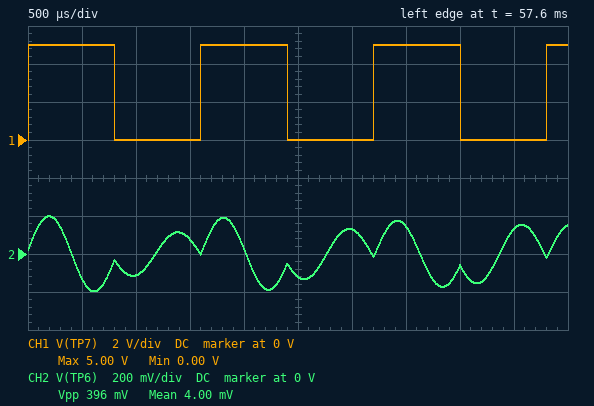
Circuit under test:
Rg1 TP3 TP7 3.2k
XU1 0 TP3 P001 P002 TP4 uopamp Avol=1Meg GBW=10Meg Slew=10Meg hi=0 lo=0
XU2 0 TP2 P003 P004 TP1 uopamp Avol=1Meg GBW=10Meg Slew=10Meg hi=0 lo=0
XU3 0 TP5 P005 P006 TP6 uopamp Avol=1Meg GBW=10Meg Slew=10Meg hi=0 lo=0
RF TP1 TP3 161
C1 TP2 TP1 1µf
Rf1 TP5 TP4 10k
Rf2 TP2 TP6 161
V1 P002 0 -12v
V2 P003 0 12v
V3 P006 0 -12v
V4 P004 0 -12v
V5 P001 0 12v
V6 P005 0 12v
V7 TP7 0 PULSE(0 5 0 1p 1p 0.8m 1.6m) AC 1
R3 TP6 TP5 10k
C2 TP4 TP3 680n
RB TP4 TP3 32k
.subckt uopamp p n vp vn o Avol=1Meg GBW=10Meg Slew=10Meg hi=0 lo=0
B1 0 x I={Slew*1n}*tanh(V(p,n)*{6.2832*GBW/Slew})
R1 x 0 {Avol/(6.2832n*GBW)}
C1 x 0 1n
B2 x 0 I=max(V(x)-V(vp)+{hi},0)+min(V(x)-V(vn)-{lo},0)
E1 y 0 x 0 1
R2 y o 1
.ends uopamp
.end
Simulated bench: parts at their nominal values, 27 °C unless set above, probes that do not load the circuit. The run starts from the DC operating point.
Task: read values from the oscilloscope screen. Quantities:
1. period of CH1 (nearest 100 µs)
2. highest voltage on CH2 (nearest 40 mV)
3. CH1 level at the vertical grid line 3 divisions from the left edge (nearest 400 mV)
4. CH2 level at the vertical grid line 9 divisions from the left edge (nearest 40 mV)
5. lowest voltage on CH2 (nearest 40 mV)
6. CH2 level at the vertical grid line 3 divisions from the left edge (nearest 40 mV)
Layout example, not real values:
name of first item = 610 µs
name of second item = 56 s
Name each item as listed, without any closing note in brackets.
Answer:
period of CH1 = 1.6 ms
highest voltage on CH2 = 200 mV
CH1 level at the vertical grid line 3 divisions from the left edge = 0 V
CH2 level at the vertical grid line 9 divisions from the left edge = 120 mV
lowest voltage on CH2 = -200 mV
CH2 level at the vertical grid line 3 divisions from the left edge = 80 mV
